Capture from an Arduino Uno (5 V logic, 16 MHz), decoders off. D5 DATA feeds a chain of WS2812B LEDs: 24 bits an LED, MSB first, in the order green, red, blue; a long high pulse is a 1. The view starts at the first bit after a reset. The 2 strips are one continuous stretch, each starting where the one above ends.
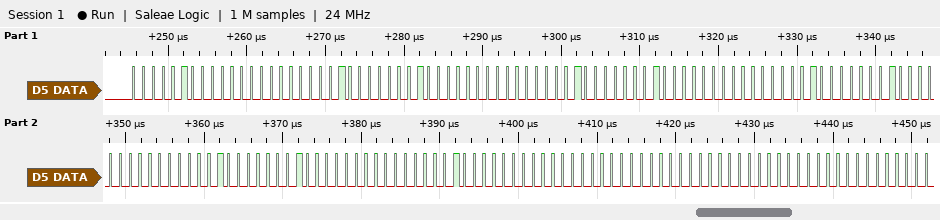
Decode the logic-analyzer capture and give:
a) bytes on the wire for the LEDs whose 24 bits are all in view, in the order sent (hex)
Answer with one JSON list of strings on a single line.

["04 00 04 04 00 04 04 00 04 04 00 04 04 00 04 00 00 00"]
